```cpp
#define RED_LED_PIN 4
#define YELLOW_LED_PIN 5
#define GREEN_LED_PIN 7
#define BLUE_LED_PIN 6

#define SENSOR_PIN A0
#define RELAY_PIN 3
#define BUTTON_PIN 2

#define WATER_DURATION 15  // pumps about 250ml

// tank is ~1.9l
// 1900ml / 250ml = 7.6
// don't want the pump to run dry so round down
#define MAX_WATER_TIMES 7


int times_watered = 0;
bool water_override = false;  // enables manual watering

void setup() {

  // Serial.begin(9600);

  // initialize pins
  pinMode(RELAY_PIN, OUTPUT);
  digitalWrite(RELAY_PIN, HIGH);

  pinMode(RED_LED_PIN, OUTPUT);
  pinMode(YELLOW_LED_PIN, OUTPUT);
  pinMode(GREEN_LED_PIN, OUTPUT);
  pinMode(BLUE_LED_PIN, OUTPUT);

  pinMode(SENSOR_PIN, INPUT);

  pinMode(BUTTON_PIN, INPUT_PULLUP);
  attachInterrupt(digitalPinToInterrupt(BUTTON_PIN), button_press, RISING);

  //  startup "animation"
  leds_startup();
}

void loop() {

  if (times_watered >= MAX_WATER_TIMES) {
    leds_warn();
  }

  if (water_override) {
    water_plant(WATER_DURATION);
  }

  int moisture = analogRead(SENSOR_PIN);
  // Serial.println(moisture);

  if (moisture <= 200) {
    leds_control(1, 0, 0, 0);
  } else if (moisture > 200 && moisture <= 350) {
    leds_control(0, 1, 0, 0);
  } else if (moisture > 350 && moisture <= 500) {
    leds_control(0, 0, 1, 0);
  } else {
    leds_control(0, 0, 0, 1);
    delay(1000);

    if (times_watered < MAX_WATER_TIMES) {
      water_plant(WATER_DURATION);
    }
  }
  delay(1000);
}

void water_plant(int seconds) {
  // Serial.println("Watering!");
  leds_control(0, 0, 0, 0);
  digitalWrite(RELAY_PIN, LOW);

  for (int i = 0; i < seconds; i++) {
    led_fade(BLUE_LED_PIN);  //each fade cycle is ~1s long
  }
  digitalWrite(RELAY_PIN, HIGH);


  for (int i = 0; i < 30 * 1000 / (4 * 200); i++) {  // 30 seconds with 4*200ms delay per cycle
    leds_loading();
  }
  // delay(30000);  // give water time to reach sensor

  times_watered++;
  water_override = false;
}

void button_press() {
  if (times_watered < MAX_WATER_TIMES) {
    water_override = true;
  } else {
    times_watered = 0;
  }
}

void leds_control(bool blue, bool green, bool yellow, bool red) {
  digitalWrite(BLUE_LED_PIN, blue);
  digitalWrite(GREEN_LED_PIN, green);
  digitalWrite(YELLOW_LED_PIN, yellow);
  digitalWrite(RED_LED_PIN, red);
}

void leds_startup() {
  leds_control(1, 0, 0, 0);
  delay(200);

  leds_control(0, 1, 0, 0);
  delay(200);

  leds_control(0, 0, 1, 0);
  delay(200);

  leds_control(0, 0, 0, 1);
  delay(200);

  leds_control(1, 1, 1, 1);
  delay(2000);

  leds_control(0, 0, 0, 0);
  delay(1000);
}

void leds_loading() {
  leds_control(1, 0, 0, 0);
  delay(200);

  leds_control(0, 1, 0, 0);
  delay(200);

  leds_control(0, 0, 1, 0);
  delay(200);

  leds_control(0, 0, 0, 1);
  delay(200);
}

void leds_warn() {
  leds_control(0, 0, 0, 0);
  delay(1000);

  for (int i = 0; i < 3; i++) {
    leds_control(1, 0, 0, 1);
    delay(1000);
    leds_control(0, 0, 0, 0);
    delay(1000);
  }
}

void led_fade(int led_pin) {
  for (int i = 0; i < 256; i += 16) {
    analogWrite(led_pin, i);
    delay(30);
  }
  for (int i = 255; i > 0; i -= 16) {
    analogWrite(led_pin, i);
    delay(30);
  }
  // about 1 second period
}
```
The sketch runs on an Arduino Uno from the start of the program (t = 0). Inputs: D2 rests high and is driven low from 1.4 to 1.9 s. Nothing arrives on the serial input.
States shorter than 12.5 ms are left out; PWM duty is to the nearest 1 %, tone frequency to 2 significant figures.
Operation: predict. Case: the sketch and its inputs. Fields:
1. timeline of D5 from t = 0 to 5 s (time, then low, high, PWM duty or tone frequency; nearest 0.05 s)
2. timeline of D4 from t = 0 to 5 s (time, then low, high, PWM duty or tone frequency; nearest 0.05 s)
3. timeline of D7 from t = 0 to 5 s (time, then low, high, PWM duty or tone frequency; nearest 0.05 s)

0 s low; 0.4 s high; 0.6 s low; 0.8 s high; 2.8 s low
0 s low; 0.6 s high; 2.8 s low
0 s low; 0.2 s high; 0.4 s low; 0.8 s high; 2.8 s low
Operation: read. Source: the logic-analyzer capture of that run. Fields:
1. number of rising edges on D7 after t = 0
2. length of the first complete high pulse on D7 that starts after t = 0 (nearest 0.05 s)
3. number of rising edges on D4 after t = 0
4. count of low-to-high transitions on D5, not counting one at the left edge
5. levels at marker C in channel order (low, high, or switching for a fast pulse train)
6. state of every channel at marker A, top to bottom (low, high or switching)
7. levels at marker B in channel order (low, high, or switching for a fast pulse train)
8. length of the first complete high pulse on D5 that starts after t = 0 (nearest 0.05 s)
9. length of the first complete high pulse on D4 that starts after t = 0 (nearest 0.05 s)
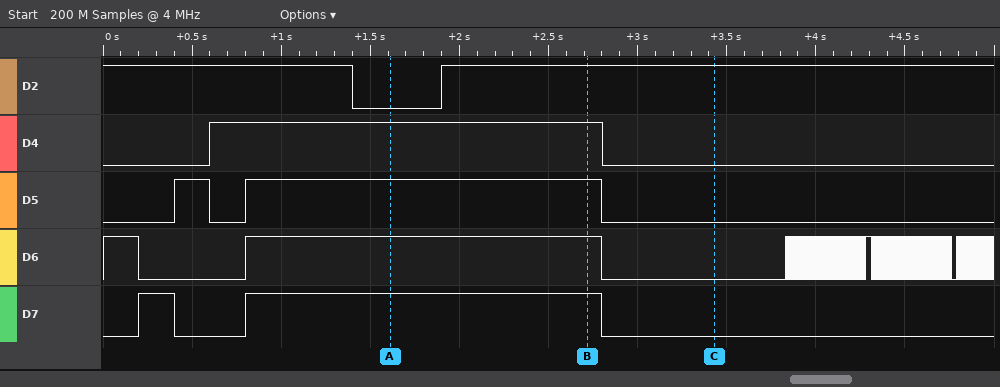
2
0.20 s
1
2
D2 high, D4 low, D5 low, D6 low, D7 low
D2 low, D4 high, D5 high, D6 high, D7 high
D2 high, D4 high, D5 high, D6 high, D7 high
0.20 s
2.20 s
